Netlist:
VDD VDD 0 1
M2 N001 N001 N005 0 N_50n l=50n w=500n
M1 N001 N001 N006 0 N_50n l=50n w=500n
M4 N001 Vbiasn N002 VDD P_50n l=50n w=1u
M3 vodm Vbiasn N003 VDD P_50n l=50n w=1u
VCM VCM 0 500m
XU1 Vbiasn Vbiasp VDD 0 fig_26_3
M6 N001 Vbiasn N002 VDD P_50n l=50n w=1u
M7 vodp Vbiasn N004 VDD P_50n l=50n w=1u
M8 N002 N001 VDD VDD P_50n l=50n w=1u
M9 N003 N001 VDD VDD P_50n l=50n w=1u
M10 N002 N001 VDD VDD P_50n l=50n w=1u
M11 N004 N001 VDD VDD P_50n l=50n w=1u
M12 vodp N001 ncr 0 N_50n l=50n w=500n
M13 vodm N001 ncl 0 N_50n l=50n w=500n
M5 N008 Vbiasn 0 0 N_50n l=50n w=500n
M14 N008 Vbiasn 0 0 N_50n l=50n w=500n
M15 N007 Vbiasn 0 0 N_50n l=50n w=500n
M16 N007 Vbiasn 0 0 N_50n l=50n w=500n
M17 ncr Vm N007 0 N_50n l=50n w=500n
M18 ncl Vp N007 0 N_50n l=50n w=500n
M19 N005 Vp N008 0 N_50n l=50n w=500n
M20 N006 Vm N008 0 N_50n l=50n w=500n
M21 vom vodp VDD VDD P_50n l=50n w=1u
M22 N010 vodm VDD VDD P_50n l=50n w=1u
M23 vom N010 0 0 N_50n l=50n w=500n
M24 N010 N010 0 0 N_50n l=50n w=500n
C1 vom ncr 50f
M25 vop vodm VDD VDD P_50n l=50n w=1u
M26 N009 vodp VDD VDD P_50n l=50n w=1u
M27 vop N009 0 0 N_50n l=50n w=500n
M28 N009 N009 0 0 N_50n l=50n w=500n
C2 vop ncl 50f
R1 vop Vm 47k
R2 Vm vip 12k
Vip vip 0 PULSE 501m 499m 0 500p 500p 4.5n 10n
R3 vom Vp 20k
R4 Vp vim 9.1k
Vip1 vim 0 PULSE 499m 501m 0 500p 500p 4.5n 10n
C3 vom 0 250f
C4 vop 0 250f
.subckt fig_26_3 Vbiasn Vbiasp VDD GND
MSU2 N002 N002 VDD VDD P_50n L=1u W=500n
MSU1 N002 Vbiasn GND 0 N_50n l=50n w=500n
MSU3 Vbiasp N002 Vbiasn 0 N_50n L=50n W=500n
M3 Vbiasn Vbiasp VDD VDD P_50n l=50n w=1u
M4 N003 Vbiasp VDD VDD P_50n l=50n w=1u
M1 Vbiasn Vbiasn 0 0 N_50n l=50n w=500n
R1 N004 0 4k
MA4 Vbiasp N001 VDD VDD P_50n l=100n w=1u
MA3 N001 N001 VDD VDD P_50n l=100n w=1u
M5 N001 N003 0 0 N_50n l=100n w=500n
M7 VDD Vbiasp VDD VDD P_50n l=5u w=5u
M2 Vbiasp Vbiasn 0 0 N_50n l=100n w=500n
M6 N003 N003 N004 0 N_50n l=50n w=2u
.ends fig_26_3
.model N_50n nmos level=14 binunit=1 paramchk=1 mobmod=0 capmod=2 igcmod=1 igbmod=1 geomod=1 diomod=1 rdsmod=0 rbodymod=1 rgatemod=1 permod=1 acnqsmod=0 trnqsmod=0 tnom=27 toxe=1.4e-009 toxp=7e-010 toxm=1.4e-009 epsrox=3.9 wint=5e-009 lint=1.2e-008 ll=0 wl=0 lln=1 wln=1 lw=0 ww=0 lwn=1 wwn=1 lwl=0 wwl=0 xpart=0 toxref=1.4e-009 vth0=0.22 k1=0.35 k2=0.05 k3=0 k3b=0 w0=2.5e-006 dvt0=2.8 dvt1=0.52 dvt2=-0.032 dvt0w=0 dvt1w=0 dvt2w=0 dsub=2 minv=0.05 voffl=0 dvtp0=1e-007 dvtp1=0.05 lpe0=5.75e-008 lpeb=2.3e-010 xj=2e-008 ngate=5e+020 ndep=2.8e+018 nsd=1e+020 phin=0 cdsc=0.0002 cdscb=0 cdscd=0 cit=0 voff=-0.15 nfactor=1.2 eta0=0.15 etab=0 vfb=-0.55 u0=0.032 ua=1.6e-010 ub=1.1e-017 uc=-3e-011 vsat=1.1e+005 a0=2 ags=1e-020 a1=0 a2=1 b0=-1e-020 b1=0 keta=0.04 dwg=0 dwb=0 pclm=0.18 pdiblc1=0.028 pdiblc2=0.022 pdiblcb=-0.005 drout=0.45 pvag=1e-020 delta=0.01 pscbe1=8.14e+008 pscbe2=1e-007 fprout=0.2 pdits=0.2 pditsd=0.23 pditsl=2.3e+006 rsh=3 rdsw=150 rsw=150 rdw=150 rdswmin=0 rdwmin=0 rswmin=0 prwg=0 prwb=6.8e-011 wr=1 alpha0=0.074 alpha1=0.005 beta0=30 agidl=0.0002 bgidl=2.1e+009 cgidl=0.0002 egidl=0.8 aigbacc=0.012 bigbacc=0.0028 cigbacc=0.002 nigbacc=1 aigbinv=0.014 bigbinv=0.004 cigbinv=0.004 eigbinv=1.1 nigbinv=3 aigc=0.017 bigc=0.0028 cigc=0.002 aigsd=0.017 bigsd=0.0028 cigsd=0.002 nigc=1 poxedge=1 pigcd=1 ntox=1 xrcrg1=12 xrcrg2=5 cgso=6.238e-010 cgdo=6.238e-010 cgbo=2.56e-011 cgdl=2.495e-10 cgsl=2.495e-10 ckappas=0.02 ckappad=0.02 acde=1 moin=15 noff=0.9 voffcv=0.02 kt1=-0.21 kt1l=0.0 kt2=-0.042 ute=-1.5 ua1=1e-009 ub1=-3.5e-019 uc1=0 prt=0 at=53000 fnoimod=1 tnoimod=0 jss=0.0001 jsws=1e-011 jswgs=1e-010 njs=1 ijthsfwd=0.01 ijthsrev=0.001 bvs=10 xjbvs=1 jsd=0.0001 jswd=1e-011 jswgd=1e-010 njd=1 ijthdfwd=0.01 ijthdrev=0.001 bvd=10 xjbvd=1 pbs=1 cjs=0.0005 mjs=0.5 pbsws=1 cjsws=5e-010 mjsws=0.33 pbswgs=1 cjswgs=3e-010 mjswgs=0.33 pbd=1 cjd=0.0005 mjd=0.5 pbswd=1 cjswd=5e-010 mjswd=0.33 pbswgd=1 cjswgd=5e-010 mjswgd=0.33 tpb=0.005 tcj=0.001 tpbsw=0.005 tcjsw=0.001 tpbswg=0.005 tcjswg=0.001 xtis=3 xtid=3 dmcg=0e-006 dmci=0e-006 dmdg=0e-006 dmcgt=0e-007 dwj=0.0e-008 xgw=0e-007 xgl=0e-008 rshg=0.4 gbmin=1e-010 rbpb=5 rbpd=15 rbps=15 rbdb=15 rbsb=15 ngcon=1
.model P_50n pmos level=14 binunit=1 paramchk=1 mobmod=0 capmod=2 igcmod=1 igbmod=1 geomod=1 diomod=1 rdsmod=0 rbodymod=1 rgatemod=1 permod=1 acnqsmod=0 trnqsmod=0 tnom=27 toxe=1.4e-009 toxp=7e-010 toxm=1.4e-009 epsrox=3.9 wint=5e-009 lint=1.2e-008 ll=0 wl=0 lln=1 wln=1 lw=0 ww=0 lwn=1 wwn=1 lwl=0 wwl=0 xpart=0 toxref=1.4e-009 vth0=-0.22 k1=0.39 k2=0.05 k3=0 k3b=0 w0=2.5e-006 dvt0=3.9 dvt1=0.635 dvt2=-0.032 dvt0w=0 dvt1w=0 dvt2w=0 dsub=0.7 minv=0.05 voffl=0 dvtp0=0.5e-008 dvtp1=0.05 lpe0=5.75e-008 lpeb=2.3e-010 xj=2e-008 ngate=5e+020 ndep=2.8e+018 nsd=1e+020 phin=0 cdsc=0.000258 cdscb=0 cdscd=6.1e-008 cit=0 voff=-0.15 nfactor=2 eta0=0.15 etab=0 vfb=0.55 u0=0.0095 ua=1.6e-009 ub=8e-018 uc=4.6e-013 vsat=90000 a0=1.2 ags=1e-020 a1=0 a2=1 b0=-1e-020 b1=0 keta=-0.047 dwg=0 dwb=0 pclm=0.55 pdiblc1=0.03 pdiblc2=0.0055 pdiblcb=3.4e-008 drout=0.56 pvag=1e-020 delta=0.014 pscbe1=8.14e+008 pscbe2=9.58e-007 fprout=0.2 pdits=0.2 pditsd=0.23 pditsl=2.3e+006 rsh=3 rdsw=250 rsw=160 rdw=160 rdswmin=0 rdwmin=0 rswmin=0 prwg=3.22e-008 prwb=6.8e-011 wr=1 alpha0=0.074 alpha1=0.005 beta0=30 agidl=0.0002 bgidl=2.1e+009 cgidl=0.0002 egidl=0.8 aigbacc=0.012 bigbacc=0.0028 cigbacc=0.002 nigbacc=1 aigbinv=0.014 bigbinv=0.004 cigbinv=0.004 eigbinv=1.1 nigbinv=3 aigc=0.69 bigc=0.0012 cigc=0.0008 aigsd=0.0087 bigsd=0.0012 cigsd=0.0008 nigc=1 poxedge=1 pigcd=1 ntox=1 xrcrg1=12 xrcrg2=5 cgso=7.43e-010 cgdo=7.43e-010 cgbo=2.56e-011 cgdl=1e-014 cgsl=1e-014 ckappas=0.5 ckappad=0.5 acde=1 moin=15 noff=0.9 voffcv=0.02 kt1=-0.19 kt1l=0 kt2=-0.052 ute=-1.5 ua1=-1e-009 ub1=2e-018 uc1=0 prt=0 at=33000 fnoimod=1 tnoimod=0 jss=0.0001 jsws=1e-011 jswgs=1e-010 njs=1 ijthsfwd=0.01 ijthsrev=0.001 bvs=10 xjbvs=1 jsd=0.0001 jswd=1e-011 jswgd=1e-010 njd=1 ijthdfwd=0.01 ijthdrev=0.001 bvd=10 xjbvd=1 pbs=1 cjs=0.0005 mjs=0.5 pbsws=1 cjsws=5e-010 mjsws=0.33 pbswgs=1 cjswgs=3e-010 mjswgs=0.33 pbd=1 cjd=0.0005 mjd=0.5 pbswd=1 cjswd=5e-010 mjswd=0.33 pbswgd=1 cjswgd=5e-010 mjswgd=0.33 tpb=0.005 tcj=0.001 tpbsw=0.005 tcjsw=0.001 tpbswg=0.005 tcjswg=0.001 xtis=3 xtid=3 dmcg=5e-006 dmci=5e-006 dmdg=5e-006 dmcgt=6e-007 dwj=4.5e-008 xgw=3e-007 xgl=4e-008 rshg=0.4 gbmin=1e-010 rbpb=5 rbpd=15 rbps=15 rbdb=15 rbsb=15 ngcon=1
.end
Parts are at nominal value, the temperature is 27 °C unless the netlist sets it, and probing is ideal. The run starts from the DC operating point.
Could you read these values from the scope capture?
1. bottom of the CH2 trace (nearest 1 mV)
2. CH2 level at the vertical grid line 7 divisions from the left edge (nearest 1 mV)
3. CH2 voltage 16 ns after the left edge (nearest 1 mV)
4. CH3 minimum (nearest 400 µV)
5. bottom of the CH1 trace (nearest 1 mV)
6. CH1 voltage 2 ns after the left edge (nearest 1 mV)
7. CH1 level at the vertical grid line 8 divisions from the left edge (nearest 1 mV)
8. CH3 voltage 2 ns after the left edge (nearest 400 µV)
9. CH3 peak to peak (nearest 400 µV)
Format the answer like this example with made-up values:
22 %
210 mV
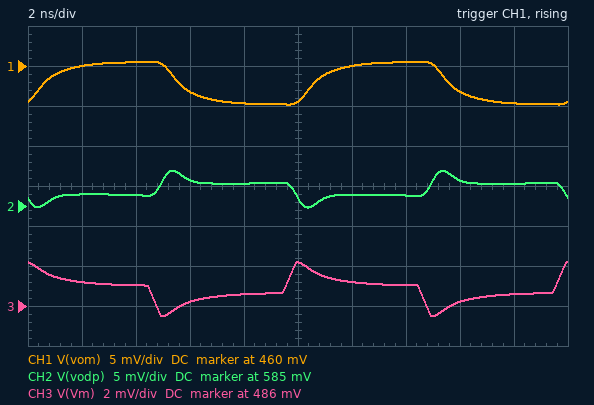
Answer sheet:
585 mV
586 mV
588 mV
485.6 mV
455 mV
460 mV
457 mV
487.2 mV
2.8 mV
